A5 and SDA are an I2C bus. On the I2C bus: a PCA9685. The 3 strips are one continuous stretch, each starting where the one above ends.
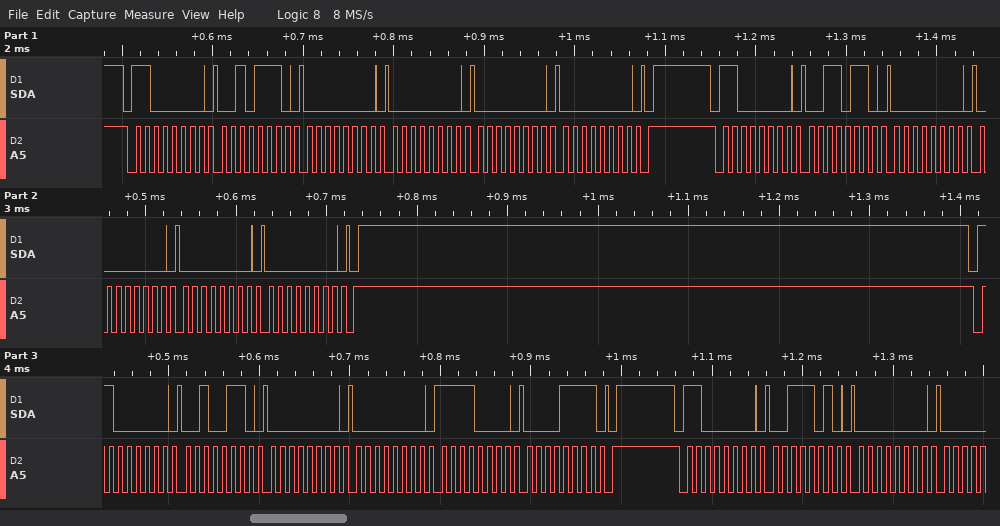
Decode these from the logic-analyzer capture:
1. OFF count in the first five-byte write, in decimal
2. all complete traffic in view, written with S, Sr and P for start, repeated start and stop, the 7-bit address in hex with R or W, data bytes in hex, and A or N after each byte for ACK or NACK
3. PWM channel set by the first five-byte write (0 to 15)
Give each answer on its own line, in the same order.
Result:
0
S 60W A 2E A 00 A 00 A 00 A 00 A P S 60W A 36 A 00 A 00 A 00 A 00 A P S 60W A 26 A 00 A 00 A F0 A 0F A P S 60W A 3A A 00 A
10
